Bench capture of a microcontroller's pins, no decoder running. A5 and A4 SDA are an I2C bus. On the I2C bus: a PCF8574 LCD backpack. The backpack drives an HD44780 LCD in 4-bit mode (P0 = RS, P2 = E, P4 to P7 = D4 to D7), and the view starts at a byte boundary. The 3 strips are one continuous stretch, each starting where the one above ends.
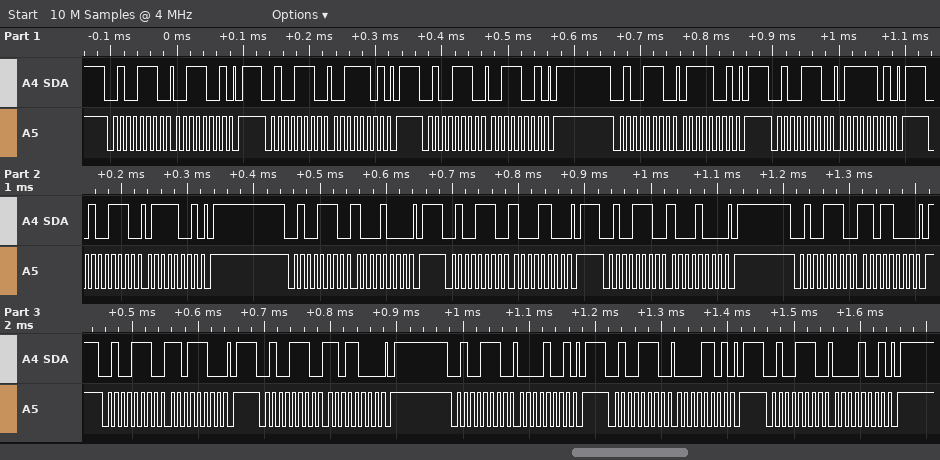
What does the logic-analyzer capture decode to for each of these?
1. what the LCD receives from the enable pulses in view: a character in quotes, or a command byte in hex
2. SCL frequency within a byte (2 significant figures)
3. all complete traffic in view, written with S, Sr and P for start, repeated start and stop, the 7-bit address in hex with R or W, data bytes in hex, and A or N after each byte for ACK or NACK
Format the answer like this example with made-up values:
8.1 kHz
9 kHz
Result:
'7' 0x8D
100 kHz
S 27W A 39 A P S 27W A 3D A P S 27W A 39 A P S 27W A 79 A P S 27W A 7D A P S 27W A 79 A P S 27W A 88 A P S 27W A 8C A P S 27W A 88 A P S 27W A D8 A P S 27W A DC A P S 27W A D8 A P S 27W A 09 A P S 27W A 0D A P S 27W A 09 A P
